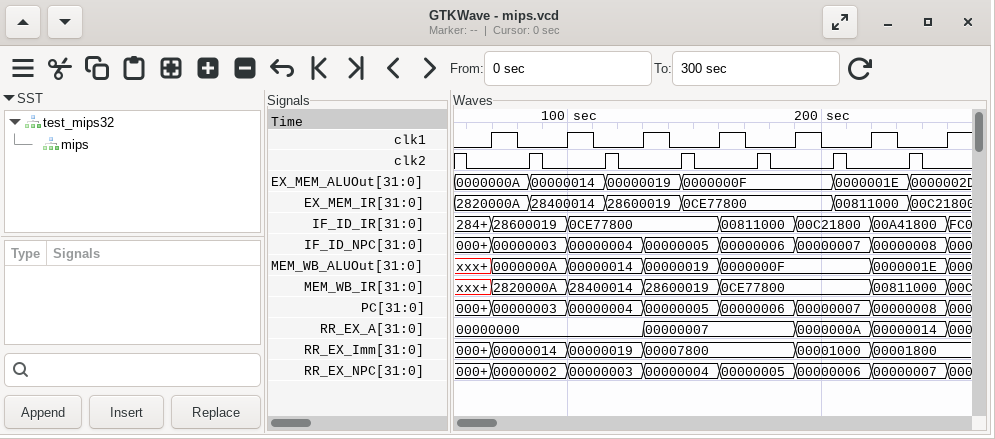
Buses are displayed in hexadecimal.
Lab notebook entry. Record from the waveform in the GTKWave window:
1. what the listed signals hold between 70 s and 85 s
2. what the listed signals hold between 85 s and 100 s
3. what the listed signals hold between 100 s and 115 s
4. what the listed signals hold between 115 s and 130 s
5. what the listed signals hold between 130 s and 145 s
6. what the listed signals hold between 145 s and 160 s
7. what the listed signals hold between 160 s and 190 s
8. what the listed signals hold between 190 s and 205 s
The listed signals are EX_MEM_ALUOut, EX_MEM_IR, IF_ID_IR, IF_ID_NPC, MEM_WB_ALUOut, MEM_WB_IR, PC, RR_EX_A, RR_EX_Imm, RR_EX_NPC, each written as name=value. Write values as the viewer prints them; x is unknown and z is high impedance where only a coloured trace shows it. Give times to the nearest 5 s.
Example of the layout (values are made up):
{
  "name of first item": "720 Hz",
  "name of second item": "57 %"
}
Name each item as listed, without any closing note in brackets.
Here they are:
{
  "what the listed signals hold between 70 s and 85 s": "EX_MEM_ALUOut=0000000A, EX_MEM_IR=2820000A, IF_ID_IR=28600019, IF_ID_NPC=00000003, MEM_WB_ALUOut=0000000A, MEM_WB_IR=2820000A, PC=00000003, RR_EX_A=00000000, RR_EX_Imm=00000014, RR_EX_NPC=00000002",
  "what the listed signals hold between 85 s and 100 s": "EX_MEM_ALUOut=00000014, EX_MEM_IR=28400014, IF_ID_IR=28600019, IF_ID_NPC=00000003, MEM_WB_ALUOut=0000000A, MEM_WB_IR=2820000A, PC=00000003, RR_EX_A=00000000, RR_EX_Imm=00000014, RR_EX_NPC=00000002",
  "what the listed signals hold between 100 s and 115 s": "EX_MEM_ALUOut=00000014, EX_MEM_IR=28400014, IF_ID_IR=0CE77800, IF_ID_NPC=00000004, MEM_WB_ALUOut=00000014, MEM_WB_IR=28400014, PC=00000004, RR_EX_A=00000000, RR_EX_Imm=00000019, RR_EX_NPC=00000003",
  "what the listed signals hold between 115 s and 130 s": "EX_MEM_ALUOut=00000019, EX_MEM_IR=28600019, IF_ID_IR=0CE77800, IF_ID_NPC=00000004, MEM_WB_ALUOut=00000014, MEM_WB_IR=28400014, PC=00000004, RR_EX_A=00000000, RR_EX_Imm=00000019, RR_EX_NPC=00000003",
  "what the listed signals hold between 130 s and 145 s": "EX_MEM_ALUOut=00000019, EX_MEM_IR=28600019, IF_ID_IR=0CE77800, IF_ID_NPC=00000005, MEM_WB_ALUOut=00000019, MEM_WB_IR=28600019, PC=00000005, RR_EX_A=00000007, RR_EX_Imm=00007800, RR_EX_NPC=00000004",
  "what the listed signals hold between 145 s and 160 s": "EX_MEM_ALUOut=0000000F, EX_MEM_IR=0CE77800, IF_ID_IR=0CE77800, IF_ID_NPC=00000005, MEM_WB_ALUOut=00000019, MEM_WB_IR=28600019, PC=00000005, RR_EX_A=00000007, RR_EX_Imm=00007800, RR_EX_NPC=00000004",
  "what the listed signals hold between 160 s and 190 s": "EX_MEM_ALUOut=0000000F, EX_MEM_IR=0CE77800, IF_ID_IR=00811000, IF_ID_NPC=00000006, MEM_WB_ALUOut=0000000F, MEM_WB_IR=0CE77800, PC=00000006, RR_EX_A=00000007, RR_EX_Imm=00007800, RR_EX_NPC=00000005",
  "what the listed signals hold between 190 s and 205 s": "EX_MEM_ALUOut=0000000F, EX_MEM_IR=0CE77800, IF_ID_IR=00C21800, IF_ID_NPC=00000007, MEM_WB_ALUOut=0000000F, MEM_WB_IR=0CE77800, PC=00000007, RR_EX_A=0000000A, RR_EX_Imm=00001000, RR_EX_NPC=00000006"
}
